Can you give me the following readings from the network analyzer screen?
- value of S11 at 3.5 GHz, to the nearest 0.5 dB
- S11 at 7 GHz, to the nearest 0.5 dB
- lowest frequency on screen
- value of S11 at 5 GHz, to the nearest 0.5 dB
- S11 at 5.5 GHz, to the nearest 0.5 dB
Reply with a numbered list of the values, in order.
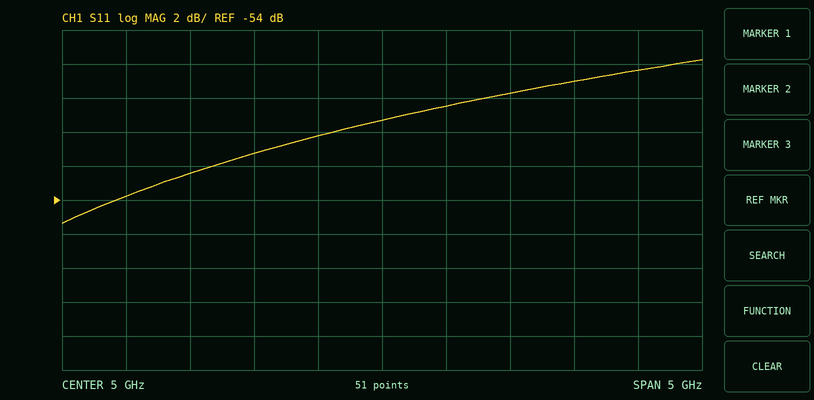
1. -52.5 dB
2. -46.5 dB
3. 2.5 GHz
4. -49.5 dB
5. -48.5 dB
